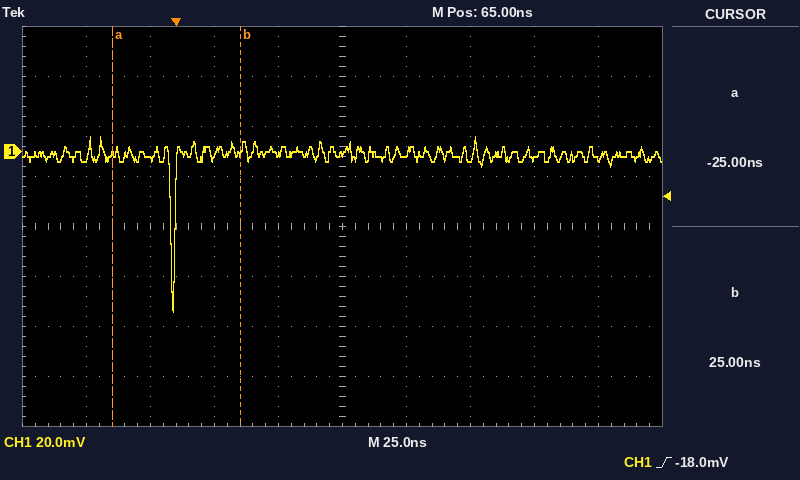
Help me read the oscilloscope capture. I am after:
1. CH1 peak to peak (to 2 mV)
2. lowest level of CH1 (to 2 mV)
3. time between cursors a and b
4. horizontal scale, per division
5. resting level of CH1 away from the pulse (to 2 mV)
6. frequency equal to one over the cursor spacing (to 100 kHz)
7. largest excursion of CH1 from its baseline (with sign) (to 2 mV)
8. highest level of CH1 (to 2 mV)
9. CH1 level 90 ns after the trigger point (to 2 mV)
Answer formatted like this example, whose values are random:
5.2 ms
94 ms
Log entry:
70 mV
-64 mV
50.0 ns
25 ns
-2 mV
20.0 MHz
-62 mV
6 mV
0 mV
